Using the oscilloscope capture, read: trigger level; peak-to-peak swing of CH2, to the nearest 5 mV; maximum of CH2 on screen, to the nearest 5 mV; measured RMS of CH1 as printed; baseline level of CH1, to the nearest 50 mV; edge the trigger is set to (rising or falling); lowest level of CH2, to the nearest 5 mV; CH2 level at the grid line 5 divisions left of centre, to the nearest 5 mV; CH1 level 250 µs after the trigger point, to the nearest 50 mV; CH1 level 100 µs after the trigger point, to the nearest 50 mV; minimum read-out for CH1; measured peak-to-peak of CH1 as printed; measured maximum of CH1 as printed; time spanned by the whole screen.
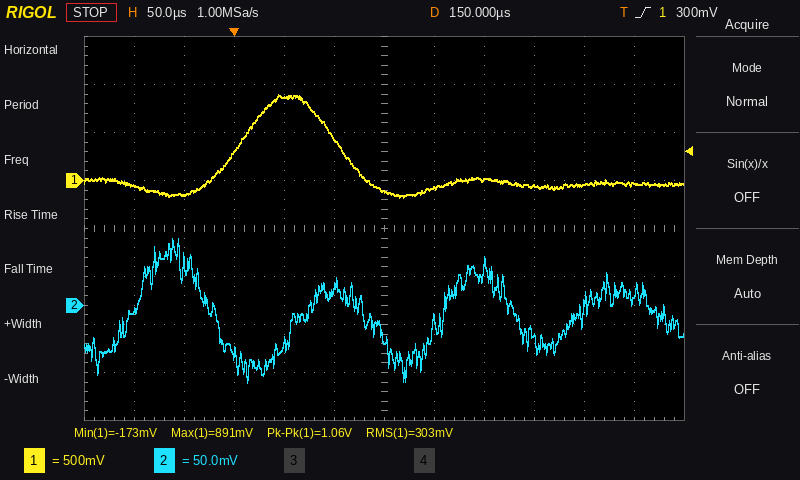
300 mV
150 mV
70 mV
303 mV
-50 mV
rising
-80 mV
-5 mV
0 mV
450 mV
-173 mV
1.06 V
891 mV
600 µs
